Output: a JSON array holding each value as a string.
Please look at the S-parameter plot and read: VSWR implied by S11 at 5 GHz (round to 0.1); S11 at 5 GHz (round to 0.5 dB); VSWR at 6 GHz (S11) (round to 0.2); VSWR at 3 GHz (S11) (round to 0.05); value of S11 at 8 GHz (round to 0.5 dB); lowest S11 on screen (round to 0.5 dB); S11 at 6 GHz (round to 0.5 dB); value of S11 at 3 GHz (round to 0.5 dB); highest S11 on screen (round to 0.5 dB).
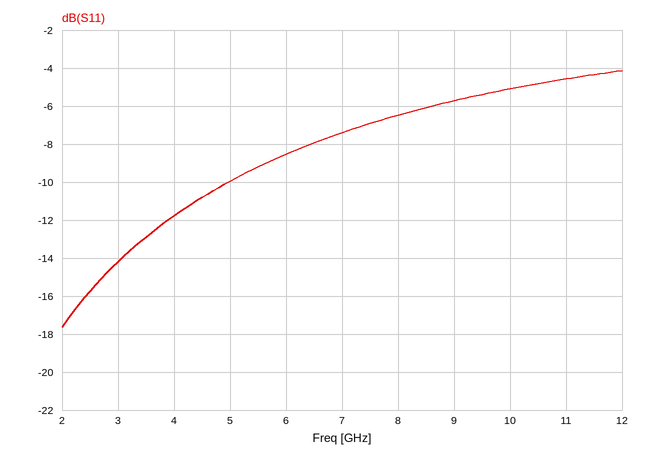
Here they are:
["1.9", "-10.0 dB", "2.2", "1.50", "-6.5 dB", "-17.5 dB", "-8.5 dB", "-14.0 dB", "-4.0 dB"]
